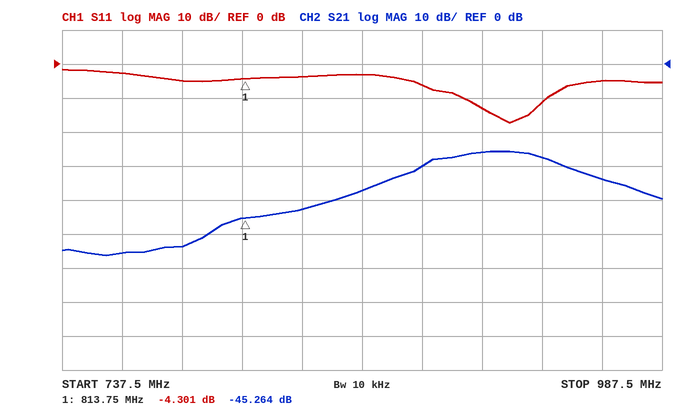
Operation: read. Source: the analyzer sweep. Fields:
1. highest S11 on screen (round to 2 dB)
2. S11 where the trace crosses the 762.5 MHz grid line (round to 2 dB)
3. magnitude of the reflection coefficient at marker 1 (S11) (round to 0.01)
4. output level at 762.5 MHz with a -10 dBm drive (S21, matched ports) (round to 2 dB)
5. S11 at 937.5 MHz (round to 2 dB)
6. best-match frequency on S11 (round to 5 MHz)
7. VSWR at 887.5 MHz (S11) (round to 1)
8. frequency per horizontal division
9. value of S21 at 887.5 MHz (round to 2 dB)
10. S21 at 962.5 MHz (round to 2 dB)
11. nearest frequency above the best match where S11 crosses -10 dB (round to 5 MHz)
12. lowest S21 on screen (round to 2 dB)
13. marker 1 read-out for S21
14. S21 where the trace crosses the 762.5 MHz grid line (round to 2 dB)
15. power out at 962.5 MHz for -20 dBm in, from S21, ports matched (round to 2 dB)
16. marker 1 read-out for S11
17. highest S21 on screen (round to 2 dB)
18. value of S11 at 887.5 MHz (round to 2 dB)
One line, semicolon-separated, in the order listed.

-2 dB; -2 dB; 0.61; -66 dBm; -12 dB; 925 MHz; 3; 25 MHz; -30 dB; -34 dB; 940 MHz; -56 dB; -45.264 dB; -56 dB; -54 dBm; -4.301 dB; -26 dB; -6 dB
